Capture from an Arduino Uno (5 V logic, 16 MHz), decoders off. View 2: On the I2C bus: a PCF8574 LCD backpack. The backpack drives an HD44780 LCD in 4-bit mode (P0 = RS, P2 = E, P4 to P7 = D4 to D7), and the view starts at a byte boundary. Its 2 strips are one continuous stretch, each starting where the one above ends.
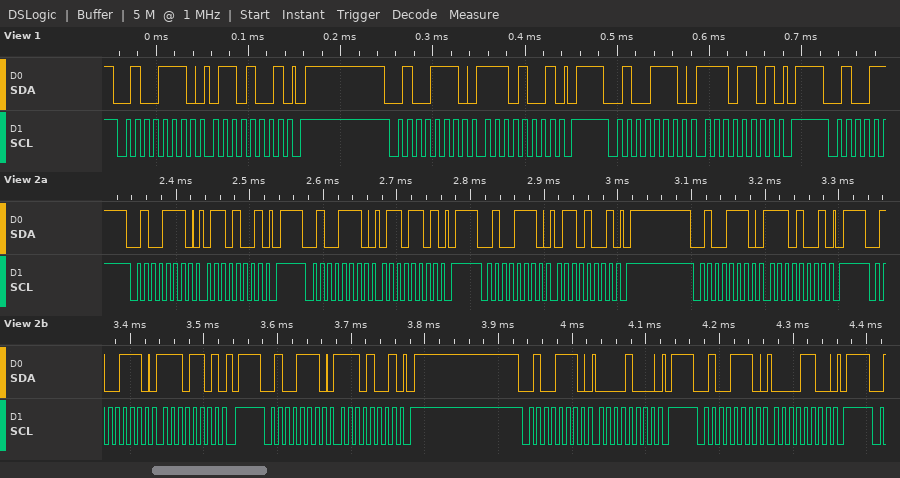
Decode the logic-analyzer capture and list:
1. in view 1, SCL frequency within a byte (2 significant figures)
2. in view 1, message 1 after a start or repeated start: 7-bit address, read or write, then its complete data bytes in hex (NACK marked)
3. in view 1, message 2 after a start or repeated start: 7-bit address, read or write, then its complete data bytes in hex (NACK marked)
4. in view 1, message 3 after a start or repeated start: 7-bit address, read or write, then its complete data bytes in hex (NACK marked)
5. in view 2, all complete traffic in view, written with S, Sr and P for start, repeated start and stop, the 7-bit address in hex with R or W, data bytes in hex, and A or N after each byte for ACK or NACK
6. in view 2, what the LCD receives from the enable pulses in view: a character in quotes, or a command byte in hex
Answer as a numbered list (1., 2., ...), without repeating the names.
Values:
1. 100 kHz
2. 0x27 write: 69
3. 0x27 write: E9
4. 0x27 write: ED
5. S 27W A 69 A P S 27W A 6D A P S 27W A 69 A P S 27W A E9 A P S 27W A ED A P S 27W A E9 A P S 27W A 08 A P S 27W A 0C A P
6. 'n'
